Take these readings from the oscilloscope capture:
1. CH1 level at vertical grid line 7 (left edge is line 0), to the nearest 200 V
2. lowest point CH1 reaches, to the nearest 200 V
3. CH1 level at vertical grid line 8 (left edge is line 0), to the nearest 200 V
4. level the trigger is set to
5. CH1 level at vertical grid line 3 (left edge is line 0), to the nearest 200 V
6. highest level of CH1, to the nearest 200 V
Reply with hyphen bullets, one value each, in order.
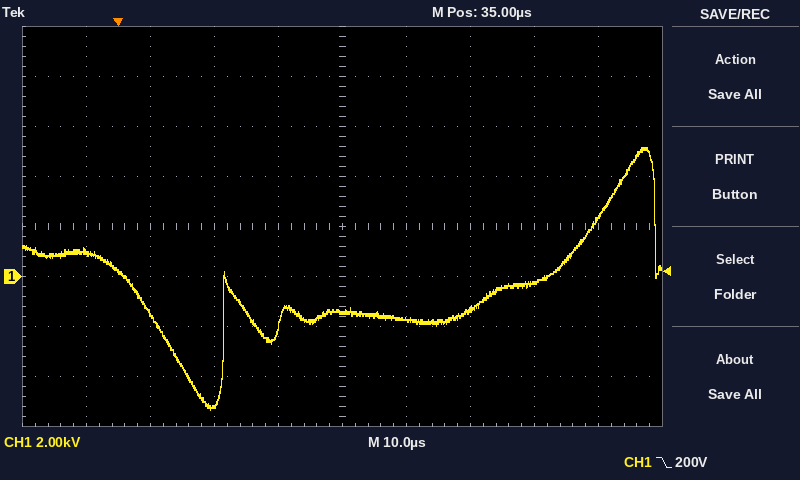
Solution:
- -1.4 kV
- -5.4 kV
- -200 V
- 200 V
- -5.2 kV
- 5.2 kV
